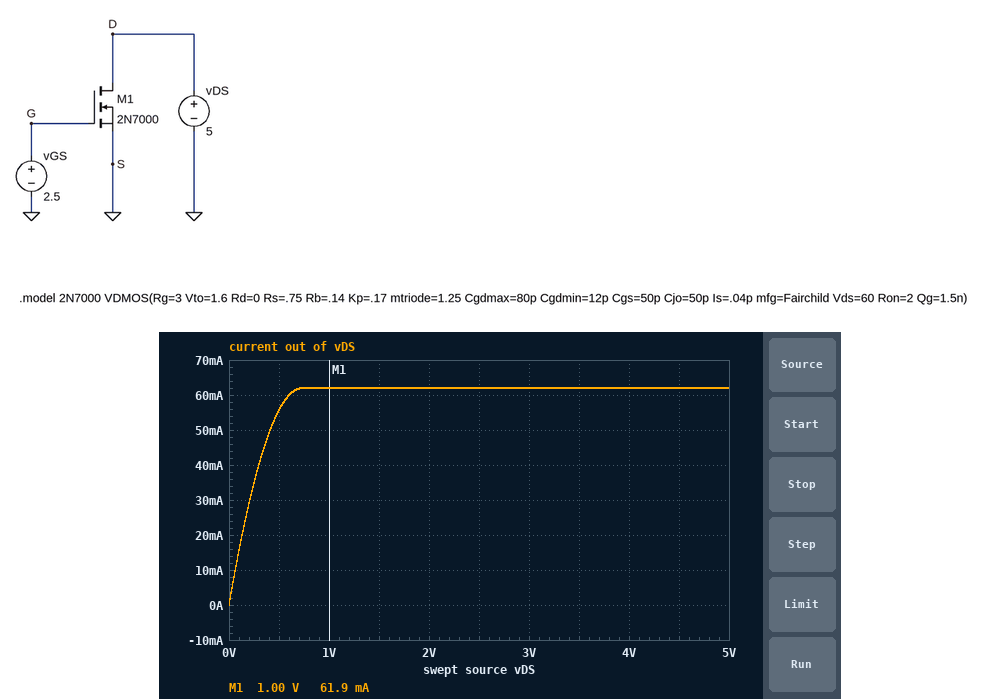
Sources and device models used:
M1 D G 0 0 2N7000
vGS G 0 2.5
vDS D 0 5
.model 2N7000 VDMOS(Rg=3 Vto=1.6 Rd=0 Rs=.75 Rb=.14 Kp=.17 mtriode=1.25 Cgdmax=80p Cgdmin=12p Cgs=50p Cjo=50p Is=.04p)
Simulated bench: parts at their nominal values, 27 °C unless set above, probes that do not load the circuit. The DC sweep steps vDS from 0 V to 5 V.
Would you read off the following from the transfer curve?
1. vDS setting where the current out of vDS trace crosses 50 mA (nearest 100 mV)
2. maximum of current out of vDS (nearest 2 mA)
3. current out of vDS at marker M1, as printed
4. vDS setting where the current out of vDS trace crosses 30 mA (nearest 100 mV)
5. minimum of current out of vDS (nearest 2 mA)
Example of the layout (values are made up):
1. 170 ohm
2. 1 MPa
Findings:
1. 400 mV
2. 62 mA
3. 61.9 mA
4. 200 mV
5. 0 A
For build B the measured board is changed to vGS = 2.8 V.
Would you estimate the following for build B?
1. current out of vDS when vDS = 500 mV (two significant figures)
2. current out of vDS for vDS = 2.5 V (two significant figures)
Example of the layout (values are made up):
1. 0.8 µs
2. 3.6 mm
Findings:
1. 81 mA
2. 110 mA
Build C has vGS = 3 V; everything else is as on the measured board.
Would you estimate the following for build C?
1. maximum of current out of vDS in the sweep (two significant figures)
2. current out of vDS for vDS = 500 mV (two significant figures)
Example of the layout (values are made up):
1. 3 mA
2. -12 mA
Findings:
1. 140 mA
2. 96 mA
